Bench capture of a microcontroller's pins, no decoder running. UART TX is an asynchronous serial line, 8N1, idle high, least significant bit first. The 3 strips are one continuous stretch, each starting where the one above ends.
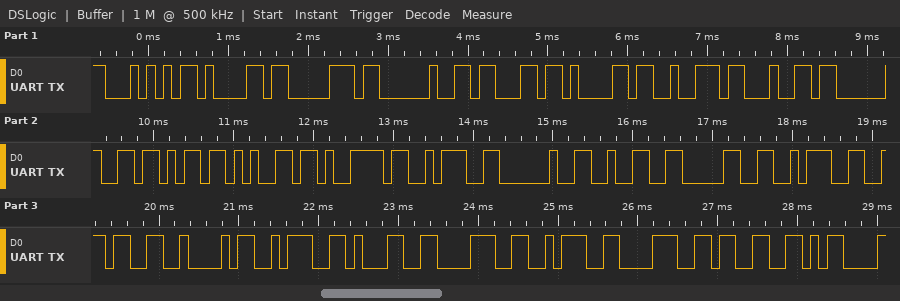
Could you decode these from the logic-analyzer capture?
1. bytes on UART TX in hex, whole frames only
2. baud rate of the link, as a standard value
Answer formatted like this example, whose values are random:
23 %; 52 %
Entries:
54 61 70 20 63 61 72 64 20 6B 65 79 3A 20 32 30 3A 36 42 3A 31 38 3A 38 33 0D; 9600 baud
